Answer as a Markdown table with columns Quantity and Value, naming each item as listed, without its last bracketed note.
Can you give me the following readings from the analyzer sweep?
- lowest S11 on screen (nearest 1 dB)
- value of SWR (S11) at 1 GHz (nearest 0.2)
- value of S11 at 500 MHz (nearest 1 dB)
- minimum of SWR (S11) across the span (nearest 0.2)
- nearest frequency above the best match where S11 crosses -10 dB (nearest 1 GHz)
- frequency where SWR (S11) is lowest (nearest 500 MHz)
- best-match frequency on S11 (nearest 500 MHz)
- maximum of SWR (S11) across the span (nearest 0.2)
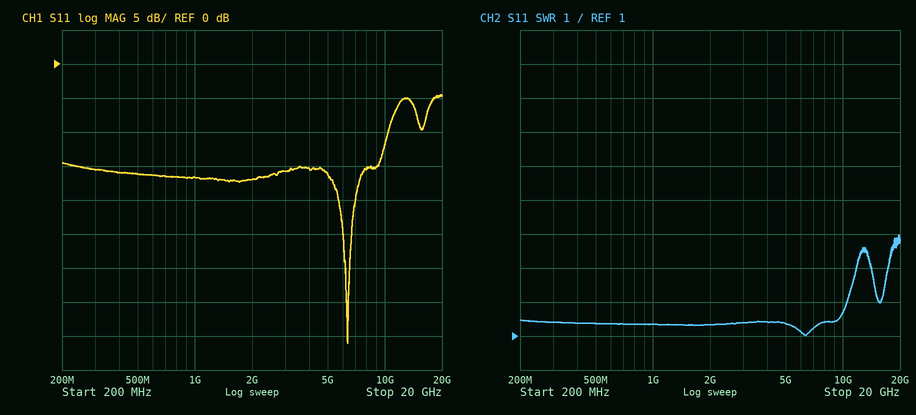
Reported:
| Quantity | Value |
|---|---|
| lowest S11 on screen | -41 dB |
| value of SWR (S11) at 1 GHz | 1.4 |
| value of S11 at 500 MHz | -16 dB |
| minimum of SWR (S11) across the span | 1.0 |
| nearest frequency above the best match where S11 crosses -10 dB | 10 GHz |
| frequency where SWR (S11) is lowest | 6.5 GHz |
| best-match frequency on S11 | 6.5 GHz |
| maximum of SWR (S11) across the span | 4.0 |
